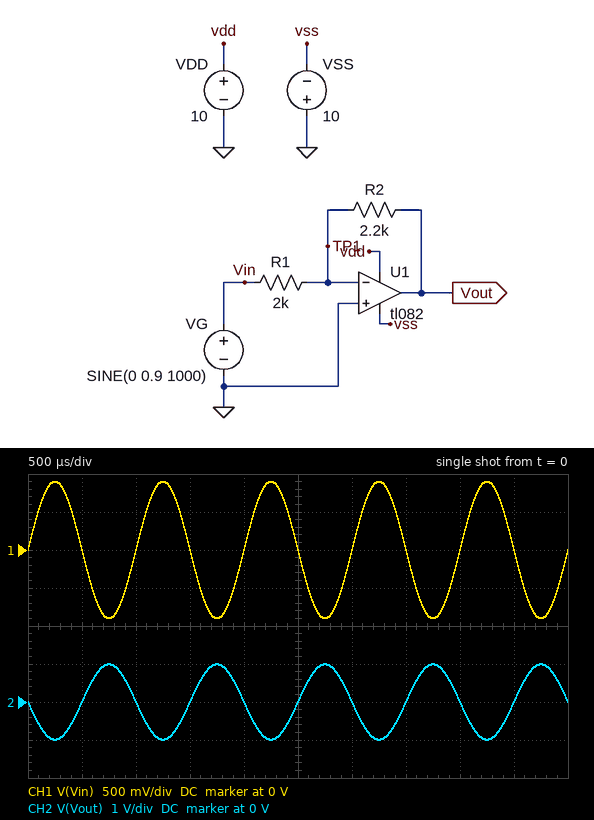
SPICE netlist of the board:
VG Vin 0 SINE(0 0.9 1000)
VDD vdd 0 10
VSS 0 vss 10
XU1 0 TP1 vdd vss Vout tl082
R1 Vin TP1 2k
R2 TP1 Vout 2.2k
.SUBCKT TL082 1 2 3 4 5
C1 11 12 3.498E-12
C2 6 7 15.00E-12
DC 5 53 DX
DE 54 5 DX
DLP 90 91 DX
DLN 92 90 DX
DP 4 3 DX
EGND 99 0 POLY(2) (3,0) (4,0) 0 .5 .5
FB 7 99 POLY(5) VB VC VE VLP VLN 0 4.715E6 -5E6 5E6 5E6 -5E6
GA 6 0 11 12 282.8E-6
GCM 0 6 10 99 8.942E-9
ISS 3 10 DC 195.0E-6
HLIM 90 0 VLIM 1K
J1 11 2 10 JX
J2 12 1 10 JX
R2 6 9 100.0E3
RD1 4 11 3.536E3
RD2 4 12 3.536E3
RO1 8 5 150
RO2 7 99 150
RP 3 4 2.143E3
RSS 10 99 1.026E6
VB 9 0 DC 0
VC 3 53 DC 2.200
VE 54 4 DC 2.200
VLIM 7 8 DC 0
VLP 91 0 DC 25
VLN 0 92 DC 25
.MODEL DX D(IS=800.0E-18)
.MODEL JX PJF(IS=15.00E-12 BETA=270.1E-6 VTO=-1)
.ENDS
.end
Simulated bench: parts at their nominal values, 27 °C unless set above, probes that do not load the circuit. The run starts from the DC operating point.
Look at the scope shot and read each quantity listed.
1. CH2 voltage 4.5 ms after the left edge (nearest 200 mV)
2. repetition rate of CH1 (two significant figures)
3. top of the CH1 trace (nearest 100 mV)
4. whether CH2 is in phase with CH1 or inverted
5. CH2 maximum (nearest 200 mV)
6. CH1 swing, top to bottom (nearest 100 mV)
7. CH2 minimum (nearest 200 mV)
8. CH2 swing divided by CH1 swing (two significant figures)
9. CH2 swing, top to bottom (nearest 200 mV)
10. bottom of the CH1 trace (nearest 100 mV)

0 V
1.0 kHz
900 mV
inverted
1.0 V
1.8 V
-1.0 V
1.1
2.0 V
-900 mV
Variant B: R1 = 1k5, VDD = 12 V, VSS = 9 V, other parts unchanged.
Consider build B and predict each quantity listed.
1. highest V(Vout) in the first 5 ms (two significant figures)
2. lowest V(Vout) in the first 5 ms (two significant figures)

1.3 V
-1.3 V
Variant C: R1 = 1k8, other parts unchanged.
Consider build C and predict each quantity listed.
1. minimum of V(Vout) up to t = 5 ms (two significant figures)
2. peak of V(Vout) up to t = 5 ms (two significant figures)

-1.1 V
1.1 V
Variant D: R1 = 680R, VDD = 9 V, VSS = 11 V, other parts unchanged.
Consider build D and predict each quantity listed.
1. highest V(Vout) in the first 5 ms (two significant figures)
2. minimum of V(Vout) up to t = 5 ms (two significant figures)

2.9 V
-2.9 V
